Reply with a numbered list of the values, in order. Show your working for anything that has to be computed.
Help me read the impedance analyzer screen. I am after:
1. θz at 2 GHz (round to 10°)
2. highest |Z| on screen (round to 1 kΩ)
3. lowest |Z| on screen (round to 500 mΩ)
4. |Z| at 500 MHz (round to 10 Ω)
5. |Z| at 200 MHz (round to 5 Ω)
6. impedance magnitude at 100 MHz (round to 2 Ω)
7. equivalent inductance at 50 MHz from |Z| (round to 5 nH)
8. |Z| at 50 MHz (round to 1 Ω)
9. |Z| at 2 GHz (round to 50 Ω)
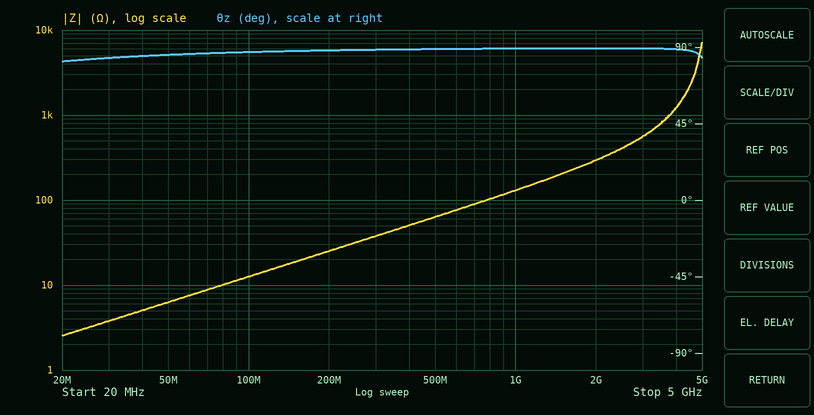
1. 90°
2. 7 kΩ
3. 2.5 Ω
4. 60 Ω
5. 25 Ω
6. 12 Ω
7. L = 6 Ω/(2π × 50 MHz) ≈ 19.1 nH, so 20 nH to the nearest 5 nH
8. 6 Ω
9. 300 Ω
